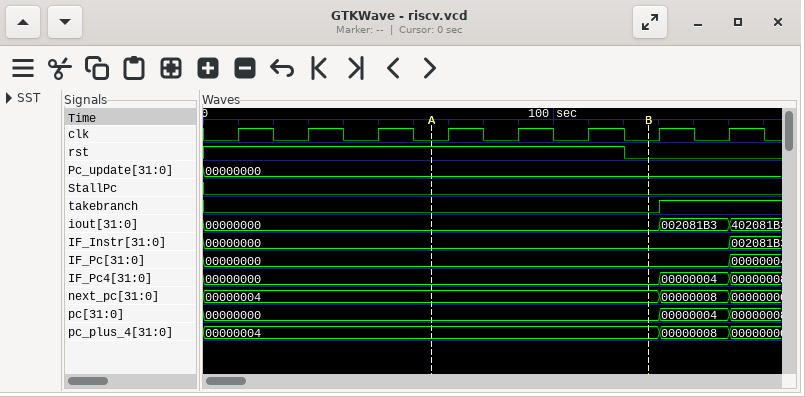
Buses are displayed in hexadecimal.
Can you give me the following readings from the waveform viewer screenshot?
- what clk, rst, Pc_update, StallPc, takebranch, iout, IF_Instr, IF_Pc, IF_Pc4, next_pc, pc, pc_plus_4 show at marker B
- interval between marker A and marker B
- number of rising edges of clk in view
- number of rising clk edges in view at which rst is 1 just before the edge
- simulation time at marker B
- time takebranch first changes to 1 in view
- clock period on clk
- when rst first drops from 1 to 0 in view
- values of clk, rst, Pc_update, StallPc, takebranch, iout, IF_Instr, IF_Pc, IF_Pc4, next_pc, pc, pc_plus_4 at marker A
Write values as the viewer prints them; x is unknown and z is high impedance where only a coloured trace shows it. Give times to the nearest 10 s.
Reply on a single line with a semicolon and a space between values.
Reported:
clk=0, rst=0, Pc_update=00000000, StallPc=0, takebranch=0, iout=00000000, IF_Instr=00000000, IF_Pc=00000000, IF_Pc4=00000000, next_pc=00000004, pc=00000000, pc_plus_4=00000004; 60 s; 8; 6; 130 s; 130 s; 20 s; 120 s; clk=0, rst=1, Pc_update=00000000, StallPc=0, takebranch=0, iout=00000000, IF_Instr=00000000, IF_Pc=00000000, IF_Pc4=00000000, next_pc=00000004, pc=00000000, pc_plus_4=00000004
